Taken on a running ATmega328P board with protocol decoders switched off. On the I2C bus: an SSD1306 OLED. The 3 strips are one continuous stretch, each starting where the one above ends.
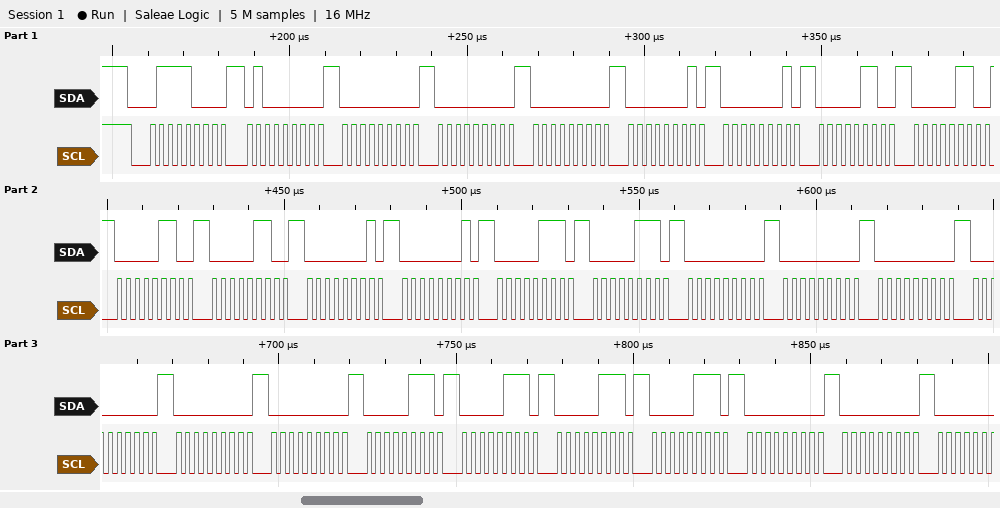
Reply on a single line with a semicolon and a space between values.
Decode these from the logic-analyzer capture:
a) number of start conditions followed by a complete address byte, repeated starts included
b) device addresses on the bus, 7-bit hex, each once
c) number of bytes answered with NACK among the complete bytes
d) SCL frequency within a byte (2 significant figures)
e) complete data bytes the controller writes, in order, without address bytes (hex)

1; 0x3C; 0; 400 kHz; 40 00 00 00 01 01 06 06 06 06 01 01 07 07 00 00 00 00 00 00 07 07 07 07 00 00
